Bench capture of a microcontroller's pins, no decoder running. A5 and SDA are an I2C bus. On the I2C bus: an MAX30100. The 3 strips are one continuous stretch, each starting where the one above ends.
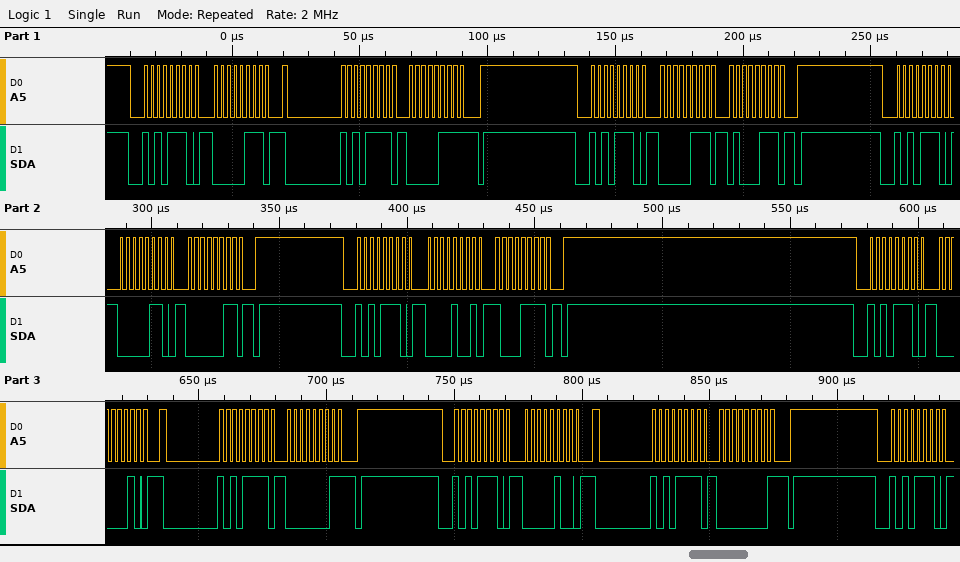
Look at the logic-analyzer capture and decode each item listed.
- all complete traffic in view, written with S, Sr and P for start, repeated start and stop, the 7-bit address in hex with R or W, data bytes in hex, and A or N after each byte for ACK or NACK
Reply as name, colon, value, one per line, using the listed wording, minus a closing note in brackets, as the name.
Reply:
all complete traffic in view, written with S, Sr and P for start, repeated start and stop, the 7-bit address in hex with R or W, data bytes in hex, and A or N after each byte for ACK or NACK: S 57W A 07 A Sr 57R A 07 N P S 57W A 07 A 47 A P S 57W A 06 A 03 A P S 57W A 09 A 8F A P S 57W A 02 A Sr 57R A 01 N P S 57W A 04 A Sr 57R A 00 N P S 57W A
